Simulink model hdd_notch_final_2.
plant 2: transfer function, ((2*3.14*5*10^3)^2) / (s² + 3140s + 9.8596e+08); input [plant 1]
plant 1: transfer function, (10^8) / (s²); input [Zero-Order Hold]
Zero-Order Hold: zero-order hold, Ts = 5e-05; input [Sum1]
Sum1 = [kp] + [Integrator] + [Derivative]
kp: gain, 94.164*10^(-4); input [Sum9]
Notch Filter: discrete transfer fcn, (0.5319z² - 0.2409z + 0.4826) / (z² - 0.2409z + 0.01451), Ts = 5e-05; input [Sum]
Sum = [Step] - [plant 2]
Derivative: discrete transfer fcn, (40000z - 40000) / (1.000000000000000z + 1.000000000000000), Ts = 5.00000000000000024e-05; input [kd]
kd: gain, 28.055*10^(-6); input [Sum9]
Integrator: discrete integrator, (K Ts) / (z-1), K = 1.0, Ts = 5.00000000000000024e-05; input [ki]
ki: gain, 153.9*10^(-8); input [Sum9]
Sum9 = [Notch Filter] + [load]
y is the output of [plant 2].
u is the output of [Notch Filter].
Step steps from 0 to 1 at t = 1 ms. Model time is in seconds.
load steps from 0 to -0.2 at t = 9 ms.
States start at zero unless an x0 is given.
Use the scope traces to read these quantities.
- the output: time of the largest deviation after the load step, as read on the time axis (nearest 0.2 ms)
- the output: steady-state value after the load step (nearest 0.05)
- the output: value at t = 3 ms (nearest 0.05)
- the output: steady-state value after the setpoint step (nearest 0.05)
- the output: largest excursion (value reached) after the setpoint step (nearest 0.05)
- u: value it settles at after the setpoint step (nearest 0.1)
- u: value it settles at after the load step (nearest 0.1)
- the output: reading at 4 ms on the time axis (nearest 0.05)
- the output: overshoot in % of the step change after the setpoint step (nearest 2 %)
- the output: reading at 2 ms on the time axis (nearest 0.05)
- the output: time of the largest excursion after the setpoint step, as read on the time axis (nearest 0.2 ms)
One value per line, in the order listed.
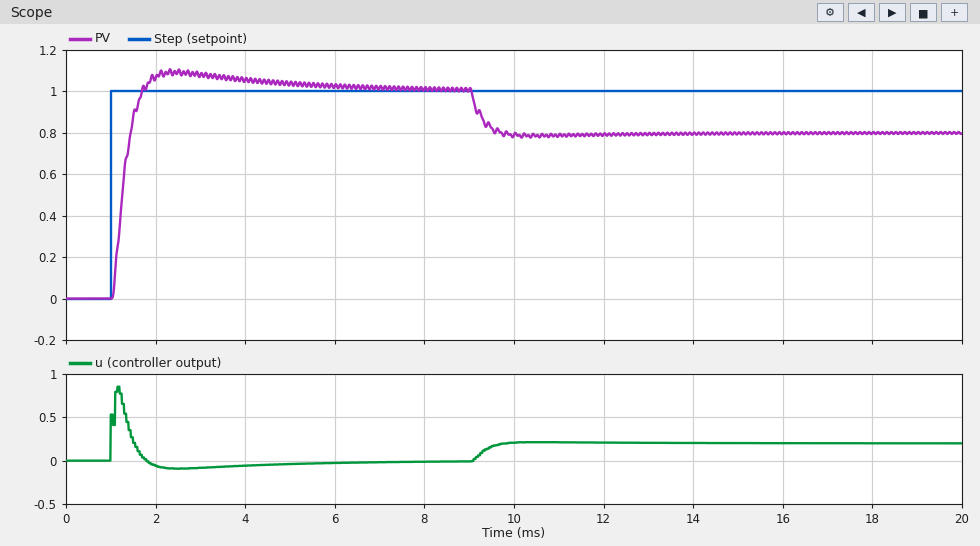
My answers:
10.2 ms
0.80
1.10
1.00
1.10
0.0
0.2
1.05
10 %
1.05
2.4 ms
